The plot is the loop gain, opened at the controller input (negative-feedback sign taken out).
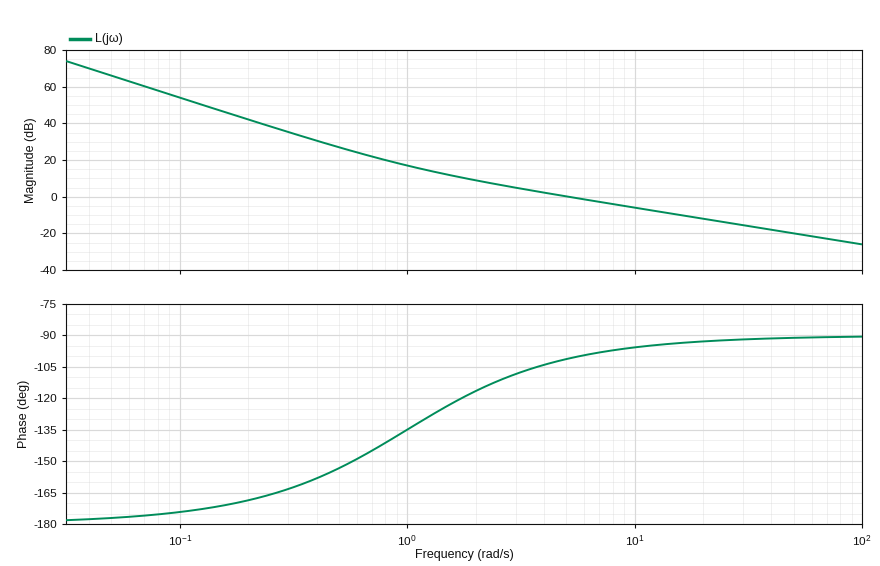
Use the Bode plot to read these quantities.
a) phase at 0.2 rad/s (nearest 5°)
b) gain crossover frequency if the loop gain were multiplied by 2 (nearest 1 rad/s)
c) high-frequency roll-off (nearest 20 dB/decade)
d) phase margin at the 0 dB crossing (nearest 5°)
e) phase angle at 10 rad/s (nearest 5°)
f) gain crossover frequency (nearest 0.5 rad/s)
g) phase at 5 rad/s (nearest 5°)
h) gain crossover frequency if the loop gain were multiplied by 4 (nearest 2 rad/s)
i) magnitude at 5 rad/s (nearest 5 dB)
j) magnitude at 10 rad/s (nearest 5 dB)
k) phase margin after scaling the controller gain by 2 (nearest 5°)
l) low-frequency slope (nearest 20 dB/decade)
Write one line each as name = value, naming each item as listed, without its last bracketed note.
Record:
phase at 0.2 rad/s = -170°
gain crossover frequency if the loop gain were multiplied by 2 = 10 rad/s
high-frequency roll-off = -20 dB/decade
phase margin at the 0 dB crossing = 80°
phase angle at 10 rad/s = -95°
gain crossover frequency = 5.0 rad/s
phase at 5 rad/s = -100°
gain crossover frequency if the loop gain were multiplied by 4 = 20 rad/s
magnitude at 5 rad/s = 0 dB
magnitude at 10 rad/s = -5 dB
phase margin after scaling the controller gain by 2 = 85°
low-frequency slope = -40 dB/decade
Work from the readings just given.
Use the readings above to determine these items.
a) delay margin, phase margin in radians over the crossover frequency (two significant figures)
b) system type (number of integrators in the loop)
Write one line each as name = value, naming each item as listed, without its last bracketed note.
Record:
delay margin, phase margin in radians over the crossover frequency = 0.28 s
system type = 2
